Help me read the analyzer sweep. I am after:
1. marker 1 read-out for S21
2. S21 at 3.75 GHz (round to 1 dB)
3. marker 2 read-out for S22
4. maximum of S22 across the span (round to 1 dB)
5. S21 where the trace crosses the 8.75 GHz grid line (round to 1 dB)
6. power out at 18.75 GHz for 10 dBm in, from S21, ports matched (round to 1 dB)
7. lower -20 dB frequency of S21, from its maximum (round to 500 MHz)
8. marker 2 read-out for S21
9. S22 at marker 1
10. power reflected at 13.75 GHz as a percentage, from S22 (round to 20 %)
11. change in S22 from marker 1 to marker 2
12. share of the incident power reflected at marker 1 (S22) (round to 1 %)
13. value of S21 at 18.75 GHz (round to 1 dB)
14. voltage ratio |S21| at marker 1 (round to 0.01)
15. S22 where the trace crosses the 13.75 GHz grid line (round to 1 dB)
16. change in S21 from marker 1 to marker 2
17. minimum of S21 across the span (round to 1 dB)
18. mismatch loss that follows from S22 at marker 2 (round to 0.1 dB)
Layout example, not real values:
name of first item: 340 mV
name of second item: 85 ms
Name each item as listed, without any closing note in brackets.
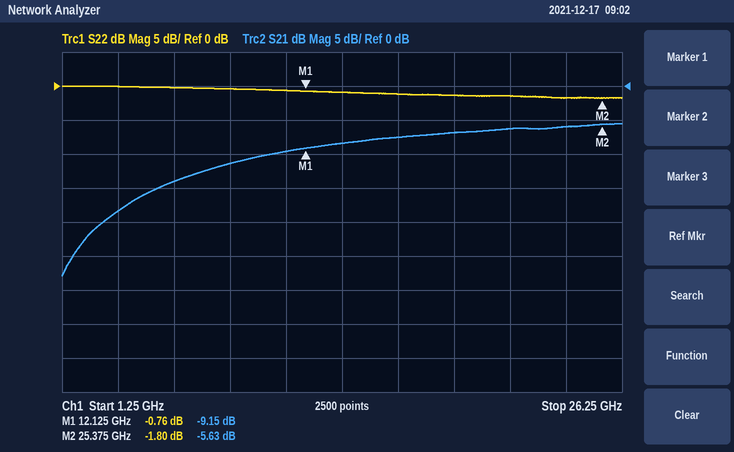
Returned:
marker 1 read-out for S21: -9.15 dB
S21 at 3.75 GHz: -18 dB
marker 2 read-out for S22: -1.80 dB
maximum of S22 across the span: 0 dB
S21 where the trace crosses the 8.75 GHz grid line: -11 dB
power out at 18.75 GHz for 10 dBm in, from S21, ports matched: 3 dBm
lower -20 dB frequency of S21, from its maximum: 1.5 GHz
marker 2 read-out for S21: -5.63 dB
S22 at marker 1: -0.76 dB
power reflected at 13.75 GHz as a percentage, from S22: 80 %
change in S22 from marker 1 to marker 2: -1.04 dB
share of the incident power reflected at marker 1 (S22): 84 %
value of S21 at 18.75 GHz: -7 dB
voltage ratio |S21| at marker 1: 0.35
S22 where the trace crosses the 13.75 GHz grid line: -1 dB
change in S21 from marker 1 to marker 2: 3.52 dB
minimum of S21 across the span: -28 dB
mismatch loss that follows from S22 at marker 2: 4.7 dB
